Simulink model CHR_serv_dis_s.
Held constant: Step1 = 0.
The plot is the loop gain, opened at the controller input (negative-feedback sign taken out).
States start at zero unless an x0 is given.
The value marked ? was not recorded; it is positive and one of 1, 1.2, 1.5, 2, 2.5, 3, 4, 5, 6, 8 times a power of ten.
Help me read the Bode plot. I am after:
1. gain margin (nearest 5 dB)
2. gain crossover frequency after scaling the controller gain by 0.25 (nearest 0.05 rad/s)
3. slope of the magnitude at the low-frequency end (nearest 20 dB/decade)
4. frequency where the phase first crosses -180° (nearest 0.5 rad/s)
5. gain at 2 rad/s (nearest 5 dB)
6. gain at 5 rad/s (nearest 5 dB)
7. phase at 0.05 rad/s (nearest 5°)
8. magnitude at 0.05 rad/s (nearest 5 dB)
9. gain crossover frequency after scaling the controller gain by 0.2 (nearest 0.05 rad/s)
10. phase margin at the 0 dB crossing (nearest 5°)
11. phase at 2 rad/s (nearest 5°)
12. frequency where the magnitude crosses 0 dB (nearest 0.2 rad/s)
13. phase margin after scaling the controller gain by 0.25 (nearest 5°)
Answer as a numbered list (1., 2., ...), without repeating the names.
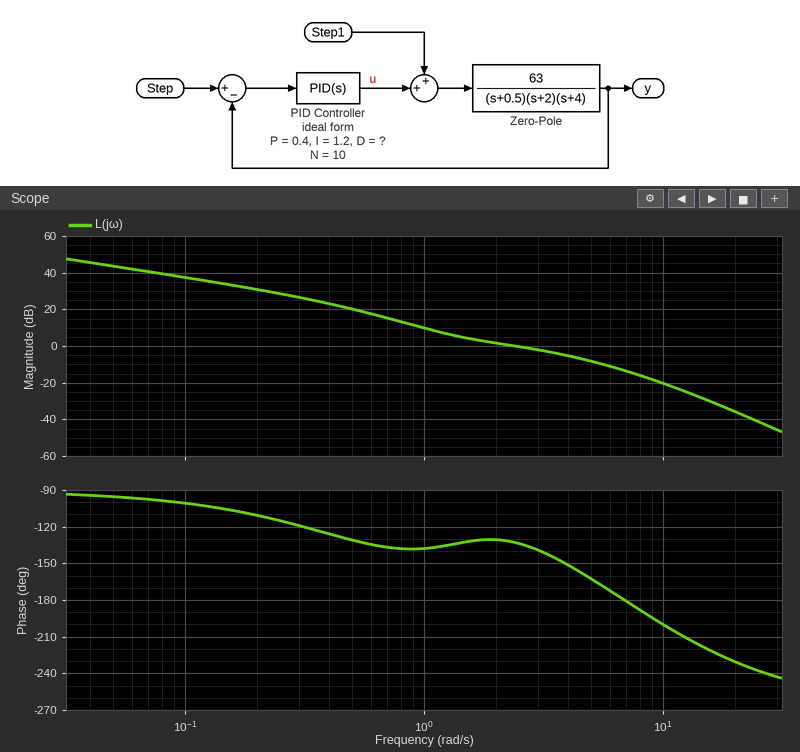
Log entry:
1. 15 dB
2. 0.85 rad/s
3. -20 dB/decade
4. 7.0 rad/s
5. 0 dB
6. -10 dB
7. -95°
8. 45 dB
9. 0.75 rad/s
10. 45°
11. -130°
12. 2.4 rad/s
13. 40°
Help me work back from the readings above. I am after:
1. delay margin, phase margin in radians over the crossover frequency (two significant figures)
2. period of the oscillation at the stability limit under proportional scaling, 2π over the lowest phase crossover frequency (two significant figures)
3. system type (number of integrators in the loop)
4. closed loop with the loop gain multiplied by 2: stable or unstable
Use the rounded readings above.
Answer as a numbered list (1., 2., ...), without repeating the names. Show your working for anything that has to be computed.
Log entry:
1. 45 × π / 180 / 2.4 = 0.33 s
2. 2π / 7 = 0.90 s
3. 1
4. stable
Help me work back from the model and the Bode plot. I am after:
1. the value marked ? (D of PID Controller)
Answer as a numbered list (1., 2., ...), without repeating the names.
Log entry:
1. 0.5
